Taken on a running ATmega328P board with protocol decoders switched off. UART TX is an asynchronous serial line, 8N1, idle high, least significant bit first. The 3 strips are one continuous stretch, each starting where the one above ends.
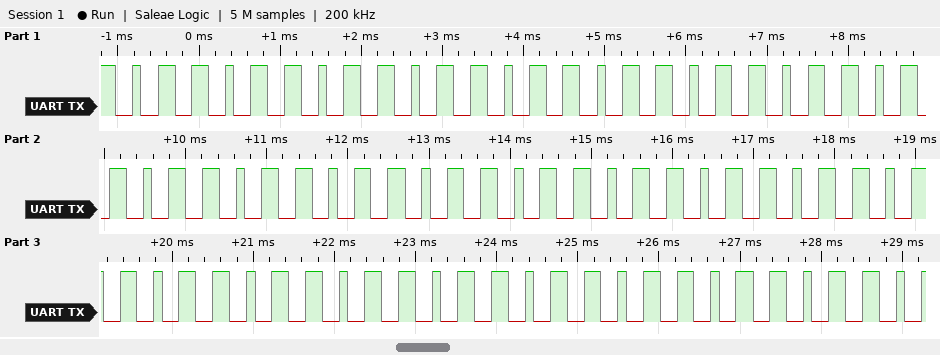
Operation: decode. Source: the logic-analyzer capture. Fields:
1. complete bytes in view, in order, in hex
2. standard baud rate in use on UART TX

0x32 0x32 0x32 0x32 0x32 0x32 0x32 0x32 0x32 0x32 0x32 0x32 0x32 0x32 0x32 0x32 0x32 0x32 0x32 0x32 0x32 0x32 0x32 0x32 0x32 0x32
9600 baud
